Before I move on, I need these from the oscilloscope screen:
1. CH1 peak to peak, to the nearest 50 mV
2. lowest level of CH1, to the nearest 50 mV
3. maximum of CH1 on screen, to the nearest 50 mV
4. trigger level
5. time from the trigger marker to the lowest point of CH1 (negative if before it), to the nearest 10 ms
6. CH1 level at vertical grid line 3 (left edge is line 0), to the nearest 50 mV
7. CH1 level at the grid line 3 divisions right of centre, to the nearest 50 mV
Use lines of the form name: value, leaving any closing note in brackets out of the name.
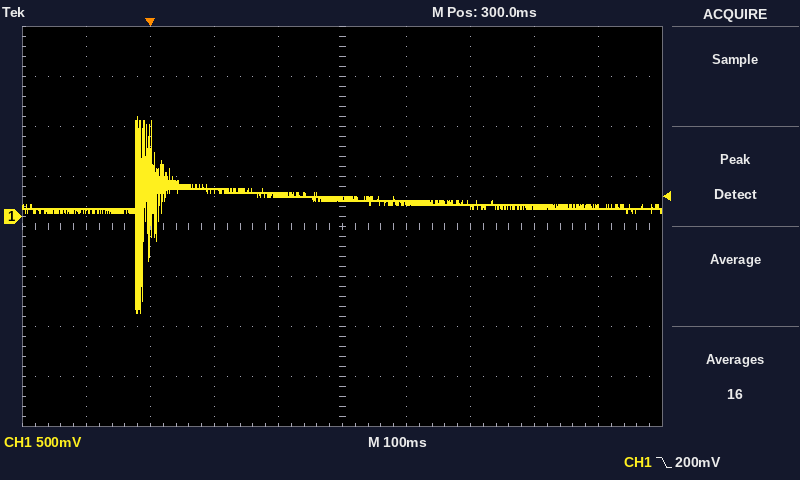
CH1 peak to peak, to the nearest 50 mV: 1.95 V
lowest level of CH1, to the nearest 50 mV: -950 mV
maximum of CH1 on screen, to the nearest 50 mV: 1.00 V
trigger level: 200 mV
time from the trigger marker to the lowest point of CH1 (negative if before it), to the nearest 10 ms: -20 ms
CH1 level at vertical grid line 3 (left edge is line 0), to the nearest 50 mV: 250 mV
CH1 level at the grid line 3 divisions right of centre, to the nearest 50 mV: 100 mV
